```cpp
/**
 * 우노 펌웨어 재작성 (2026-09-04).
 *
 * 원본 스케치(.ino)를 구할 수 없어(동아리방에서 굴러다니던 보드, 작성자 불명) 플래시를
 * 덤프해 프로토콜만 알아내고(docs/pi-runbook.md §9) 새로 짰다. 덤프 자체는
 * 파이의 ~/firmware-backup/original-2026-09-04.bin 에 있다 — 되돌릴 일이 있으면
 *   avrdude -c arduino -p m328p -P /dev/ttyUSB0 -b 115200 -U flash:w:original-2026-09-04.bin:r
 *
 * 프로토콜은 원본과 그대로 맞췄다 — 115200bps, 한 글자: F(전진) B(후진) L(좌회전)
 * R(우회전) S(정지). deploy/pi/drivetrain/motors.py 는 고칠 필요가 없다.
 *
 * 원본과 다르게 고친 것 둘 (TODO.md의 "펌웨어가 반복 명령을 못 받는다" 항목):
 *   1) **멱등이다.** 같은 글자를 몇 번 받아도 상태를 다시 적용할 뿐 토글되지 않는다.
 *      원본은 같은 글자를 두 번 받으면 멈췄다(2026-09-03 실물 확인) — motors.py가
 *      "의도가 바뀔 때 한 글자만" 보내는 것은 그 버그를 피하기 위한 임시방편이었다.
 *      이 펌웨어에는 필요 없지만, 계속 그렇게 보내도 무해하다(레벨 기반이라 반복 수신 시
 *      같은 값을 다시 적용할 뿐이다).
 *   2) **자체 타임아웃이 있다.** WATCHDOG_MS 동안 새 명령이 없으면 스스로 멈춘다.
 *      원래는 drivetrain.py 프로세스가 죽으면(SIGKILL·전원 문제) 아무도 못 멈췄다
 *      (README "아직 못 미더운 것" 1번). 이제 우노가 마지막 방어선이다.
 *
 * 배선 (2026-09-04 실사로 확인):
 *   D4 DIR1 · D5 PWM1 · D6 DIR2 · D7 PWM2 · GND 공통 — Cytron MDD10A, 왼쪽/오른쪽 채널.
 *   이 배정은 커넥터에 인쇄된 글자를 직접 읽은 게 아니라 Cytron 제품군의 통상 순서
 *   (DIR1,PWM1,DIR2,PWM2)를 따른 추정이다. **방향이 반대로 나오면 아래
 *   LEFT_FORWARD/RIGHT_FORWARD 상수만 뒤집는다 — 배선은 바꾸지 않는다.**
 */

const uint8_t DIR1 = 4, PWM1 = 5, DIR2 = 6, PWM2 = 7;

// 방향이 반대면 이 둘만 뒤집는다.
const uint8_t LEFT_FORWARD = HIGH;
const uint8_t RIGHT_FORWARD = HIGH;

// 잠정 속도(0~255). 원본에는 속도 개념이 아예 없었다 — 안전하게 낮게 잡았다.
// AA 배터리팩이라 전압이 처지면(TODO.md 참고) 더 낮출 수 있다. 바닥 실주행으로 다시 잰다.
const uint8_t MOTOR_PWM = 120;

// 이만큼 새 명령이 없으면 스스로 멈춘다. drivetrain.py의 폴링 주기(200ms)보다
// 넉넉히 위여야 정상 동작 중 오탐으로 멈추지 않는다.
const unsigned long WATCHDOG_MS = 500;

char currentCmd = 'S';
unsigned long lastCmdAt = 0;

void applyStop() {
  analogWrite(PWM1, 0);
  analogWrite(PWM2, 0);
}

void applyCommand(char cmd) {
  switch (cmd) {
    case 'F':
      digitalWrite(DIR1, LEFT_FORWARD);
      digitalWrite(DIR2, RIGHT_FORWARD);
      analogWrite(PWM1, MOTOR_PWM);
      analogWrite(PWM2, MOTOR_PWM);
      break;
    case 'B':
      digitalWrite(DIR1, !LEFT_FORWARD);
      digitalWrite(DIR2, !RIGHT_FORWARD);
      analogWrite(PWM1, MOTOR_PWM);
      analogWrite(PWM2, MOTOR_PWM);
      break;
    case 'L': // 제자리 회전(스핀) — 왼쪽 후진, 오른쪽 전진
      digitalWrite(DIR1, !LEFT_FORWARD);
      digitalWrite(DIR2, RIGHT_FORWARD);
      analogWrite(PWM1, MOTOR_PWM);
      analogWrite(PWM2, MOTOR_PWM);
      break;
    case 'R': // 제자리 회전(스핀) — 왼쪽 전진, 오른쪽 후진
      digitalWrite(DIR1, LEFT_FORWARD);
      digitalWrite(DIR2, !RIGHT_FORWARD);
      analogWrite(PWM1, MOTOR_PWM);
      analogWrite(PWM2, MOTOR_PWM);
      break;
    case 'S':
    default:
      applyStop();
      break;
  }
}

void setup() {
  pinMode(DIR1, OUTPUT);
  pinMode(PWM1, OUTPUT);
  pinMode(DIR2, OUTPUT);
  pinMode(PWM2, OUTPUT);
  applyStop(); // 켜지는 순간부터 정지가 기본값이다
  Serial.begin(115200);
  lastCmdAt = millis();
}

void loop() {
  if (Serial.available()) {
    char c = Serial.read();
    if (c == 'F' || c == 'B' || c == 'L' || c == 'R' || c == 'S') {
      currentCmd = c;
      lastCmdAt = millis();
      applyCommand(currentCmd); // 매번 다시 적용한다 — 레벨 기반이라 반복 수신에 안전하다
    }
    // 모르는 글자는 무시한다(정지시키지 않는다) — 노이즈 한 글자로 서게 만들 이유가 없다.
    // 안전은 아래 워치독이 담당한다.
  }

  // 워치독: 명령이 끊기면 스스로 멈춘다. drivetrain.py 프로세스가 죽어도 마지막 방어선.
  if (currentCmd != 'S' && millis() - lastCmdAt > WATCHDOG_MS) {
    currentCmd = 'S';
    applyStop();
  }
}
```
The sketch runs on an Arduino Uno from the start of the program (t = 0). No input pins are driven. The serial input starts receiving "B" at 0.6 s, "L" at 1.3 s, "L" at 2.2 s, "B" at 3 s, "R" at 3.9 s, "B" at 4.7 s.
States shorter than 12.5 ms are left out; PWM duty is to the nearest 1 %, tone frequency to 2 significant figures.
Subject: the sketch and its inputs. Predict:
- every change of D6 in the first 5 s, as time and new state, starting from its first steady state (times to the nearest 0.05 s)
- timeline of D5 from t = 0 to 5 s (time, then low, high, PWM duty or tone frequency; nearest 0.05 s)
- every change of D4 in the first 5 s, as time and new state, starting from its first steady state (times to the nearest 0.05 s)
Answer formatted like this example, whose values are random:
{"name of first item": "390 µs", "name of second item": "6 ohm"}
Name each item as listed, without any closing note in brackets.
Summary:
{"every change of D6 in the first 5 s, as time and new state, starting from its first steady state": "0 s low; 1.3 s high; 3 s low", "timeline of D5 from t = 0 to 5 s": "0 s low; 0.6 s PWM 47 %; 1.1 s low; 1.3 s PWM 47 %; 1.8 s low; 2.2 s PWM 47 %; 2.7 s low; 3 s PWM 47 %; 3.5 s low; 3.9 s PWM 47 %; 4.4 s low; 4.7 s PWM 47 %", "every change of D4 in the first 5 s, as time and new state, starting from its first steady state": "0 s low; 3.9 s high; 4.7 s low"}
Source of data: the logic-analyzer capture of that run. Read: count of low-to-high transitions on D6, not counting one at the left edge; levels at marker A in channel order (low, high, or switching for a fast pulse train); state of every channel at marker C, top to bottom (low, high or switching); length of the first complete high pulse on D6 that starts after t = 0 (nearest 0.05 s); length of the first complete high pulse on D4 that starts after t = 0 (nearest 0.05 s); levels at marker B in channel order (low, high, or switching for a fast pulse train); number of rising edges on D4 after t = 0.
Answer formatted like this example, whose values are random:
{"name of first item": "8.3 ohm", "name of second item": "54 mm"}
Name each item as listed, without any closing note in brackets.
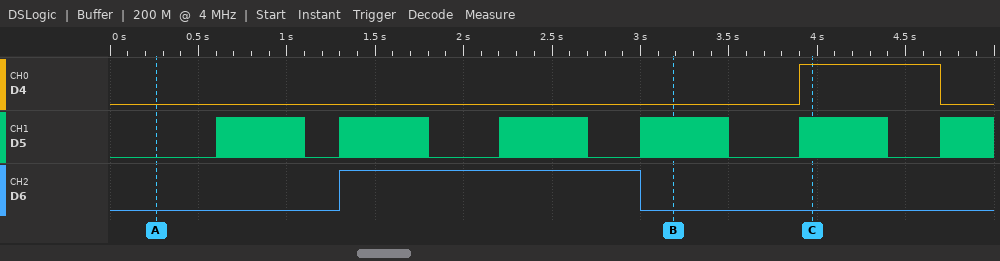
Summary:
{"count of low-to-high transitions on D6, not counting one at the left edge": "1", "levels at marker A in channel order": "D4 low, D5 low, D6 low", "state of every channel at marker C, top to bottom": "D4 high, D5 switching, D6 low", "length of the first complete high pulse on D6 that starts after t = 0": "1.70 s", "length of the first complete high pulse on D4 that starts after t = 0": "0.80 s", "levels at marker B in channel order": "D4 low, D5 switching, D6 low", "number of rising edges on D4 after t = 0": "1"}
